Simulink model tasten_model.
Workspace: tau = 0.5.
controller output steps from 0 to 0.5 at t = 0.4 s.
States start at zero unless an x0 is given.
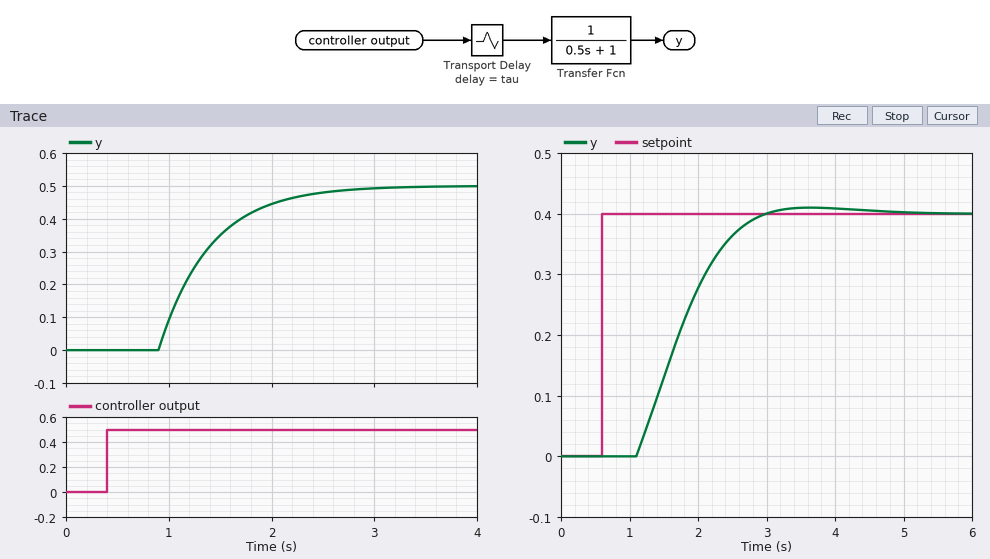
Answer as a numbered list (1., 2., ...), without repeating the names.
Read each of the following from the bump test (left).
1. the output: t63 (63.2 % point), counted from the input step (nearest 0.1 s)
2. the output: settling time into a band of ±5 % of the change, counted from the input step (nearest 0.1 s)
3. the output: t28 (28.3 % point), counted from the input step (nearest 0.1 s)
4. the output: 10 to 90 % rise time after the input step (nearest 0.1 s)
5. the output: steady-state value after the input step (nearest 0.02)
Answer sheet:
1. 1.0 s
2. 2.0 s
3. 0.7 s
4. 1.1 s
5. 0.50
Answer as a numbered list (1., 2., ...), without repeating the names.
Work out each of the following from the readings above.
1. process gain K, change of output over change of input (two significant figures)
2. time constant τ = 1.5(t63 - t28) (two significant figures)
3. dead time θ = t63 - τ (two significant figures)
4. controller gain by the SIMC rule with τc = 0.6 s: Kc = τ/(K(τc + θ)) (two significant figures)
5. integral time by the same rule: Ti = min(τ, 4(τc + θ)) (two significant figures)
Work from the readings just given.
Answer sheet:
1. 1.0
2. 0.45 s
3. 0.55 s
4. 0.39
5. 0.45 s
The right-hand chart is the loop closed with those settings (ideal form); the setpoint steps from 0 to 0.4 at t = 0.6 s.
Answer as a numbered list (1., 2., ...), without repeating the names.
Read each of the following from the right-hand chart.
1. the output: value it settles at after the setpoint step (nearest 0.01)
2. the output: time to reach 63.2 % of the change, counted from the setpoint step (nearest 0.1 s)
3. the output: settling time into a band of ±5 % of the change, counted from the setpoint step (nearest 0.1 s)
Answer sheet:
1. 0.40
2. 1.3 s
3. 2.1 s
